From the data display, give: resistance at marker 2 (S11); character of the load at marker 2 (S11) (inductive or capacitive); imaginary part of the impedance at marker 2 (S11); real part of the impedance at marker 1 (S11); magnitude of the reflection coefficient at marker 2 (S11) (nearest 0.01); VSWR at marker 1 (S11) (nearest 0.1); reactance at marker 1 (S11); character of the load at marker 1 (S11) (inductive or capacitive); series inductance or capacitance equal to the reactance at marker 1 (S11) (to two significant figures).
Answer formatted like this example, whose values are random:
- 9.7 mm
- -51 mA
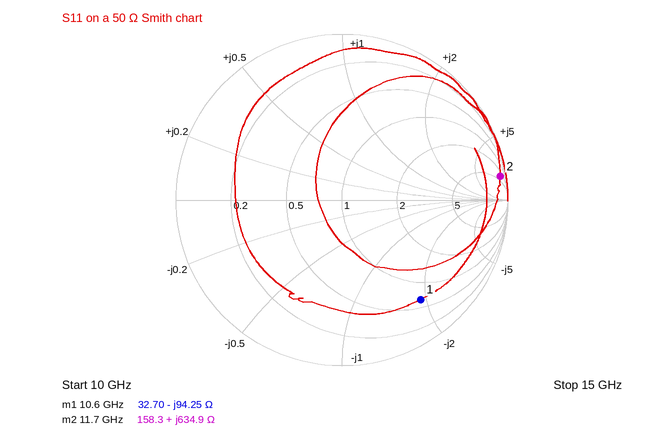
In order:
- 158.3 Ω
- inductive
- +634.9 Ω
- 32.70 Ω
- 0.96
- 7.5
- -94.25 Ω
- capacitive
- 160 fF
